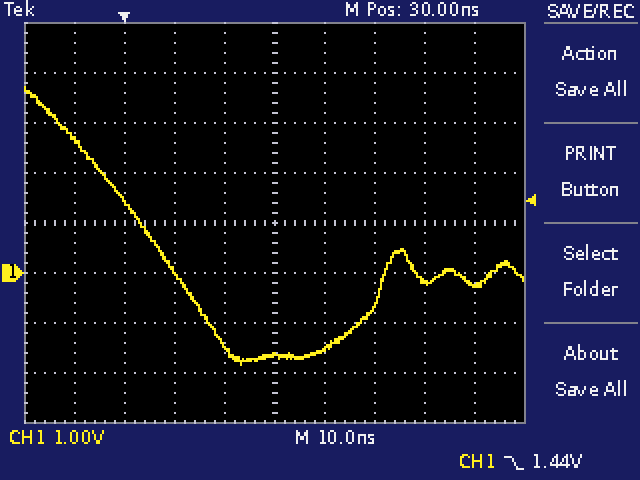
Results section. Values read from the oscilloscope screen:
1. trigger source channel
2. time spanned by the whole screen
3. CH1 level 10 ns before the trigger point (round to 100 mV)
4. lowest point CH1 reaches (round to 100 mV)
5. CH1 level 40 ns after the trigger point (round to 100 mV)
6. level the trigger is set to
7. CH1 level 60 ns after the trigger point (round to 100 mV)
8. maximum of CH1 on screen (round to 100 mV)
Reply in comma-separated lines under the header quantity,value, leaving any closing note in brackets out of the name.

quantity,value
trigger source channel,CH1
time spanned by the whole screen,100 ns
CH1 level 10 ns before the trigger point,2.7 V
lowest point CH1 reaches,-1.8 V
CH1 level 40 ns after the trigger point,-1.5 V
level the trigger is set to,1.44 V
CH1 level 60 ns after the trigger point,-200 mV
maximum of CH1 on screen,3.7 V
